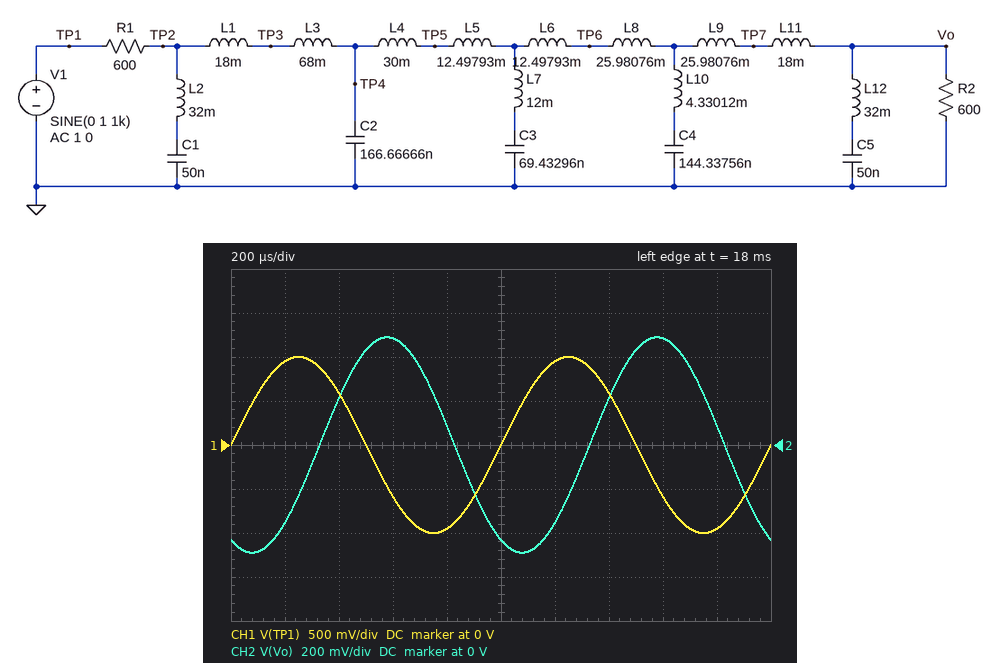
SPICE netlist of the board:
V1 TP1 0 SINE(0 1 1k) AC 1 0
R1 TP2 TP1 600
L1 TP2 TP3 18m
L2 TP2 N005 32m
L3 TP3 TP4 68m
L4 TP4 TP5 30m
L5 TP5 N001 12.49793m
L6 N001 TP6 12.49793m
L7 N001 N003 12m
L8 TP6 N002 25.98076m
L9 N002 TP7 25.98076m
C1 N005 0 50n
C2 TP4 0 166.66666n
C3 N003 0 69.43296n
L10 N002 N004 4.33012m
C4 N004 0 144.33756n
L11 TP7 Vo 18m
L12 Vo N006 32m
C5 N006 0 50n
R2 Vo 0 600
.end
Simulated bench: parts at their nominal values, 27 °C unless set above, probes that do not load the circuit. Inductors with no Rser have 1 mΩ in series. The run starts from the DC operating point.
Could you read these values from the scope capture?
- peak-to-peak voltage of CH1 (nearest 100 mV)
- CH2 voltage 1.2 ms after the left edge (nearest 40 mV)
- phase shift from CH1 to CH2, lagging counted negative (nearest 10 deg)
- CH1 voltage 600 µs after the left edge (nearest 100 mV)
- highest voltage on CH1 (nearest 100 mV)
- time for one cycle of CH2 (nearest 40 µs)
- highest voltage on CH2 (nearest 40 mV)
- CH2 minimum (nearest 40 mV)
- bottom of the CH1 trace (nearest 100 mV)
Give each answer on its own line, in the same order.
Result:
2.0 V
-360 mV
-120 deg
-600 mV
1.0 V
1.00 ms
480 mV
-480 mV
-1.0 V
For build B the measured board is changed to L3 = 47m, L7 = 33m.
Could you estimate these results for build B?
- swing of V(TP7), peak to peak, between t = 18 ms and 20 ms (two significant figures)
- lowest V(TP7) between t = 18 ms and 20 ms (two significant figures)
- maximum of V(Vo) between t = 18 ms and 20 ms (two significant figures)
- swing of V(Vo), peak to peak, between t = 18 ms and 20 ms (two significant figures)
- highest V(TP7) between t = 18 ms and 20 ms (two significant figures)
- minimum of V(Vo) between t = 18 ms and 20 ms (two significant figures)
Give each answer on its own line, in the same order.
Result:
980 mV
-490 mV
500 mV
1.0 V
490 mV
-500 mV
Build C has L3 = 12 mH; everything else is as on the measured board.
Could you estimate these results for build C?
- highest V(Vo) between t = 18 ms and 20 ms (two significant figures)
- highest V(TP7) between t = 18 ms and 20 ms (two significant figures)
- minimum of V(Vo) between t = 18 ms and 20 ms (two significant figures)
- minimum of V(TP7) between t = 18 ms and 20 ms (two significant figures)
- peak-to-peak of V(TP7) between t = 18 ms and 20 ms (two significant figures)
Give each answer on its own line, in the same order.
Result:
500 mV
490 mV
-500 mV
-490 mV
980 mV
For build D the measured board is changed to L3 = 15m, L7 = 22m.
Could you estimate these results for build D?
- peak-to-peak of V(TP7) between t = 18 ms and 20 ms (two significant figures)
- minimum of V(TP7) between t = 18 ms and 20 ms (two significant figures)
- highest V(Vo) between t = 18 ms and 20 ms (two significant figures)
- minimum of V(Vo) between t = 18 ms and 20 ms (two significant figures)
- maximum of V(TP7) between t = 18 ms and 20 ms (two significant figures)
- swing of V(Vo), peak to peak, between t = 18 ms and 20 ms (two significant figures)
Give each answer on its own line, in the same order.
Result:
980 mV
-490 mV
500 mV
-500 mV
490 mV
1.0 V
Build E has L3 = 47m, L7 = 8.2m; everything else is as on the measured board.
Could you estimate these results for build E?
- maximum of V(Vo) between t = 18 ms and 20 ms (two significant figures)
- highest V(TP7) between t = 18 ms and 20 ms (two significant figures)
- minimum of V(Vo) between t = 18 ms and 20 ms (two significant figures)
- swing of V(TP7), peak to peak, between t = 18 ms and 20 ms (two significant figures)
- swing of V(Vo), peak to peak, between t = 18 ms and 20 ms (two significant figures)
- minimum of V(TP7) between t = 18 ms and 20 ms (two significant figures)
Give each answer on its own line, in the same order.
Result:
500 mV
490 mV
-500 mV
980 mV
1.0 V
-490 mV
